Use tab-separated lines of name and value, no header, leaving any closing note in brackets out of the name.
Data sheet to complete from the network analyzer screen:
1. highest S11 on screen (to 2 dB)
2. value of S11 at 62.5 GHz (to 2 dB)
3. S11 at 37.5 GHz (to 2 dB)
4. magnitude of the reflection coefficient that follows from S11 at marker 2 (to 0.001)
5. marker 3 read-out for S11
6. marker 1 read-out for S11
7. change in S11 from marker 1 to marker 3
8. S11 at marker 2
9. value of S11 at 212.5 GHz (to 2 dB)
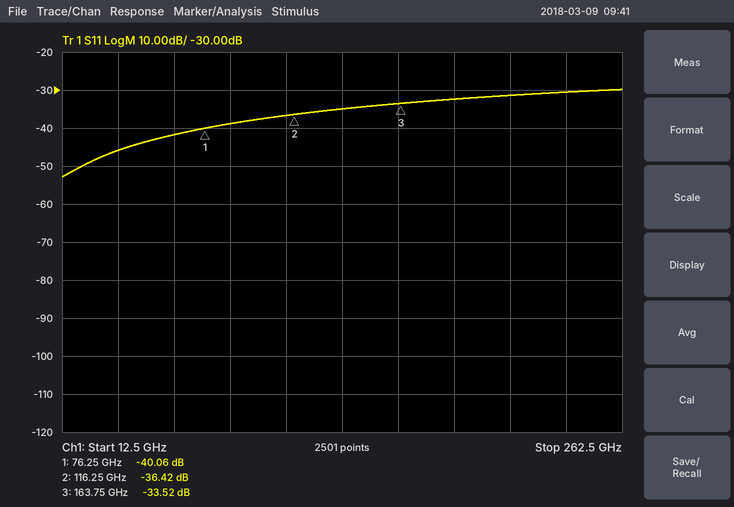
highest S11 on screen	-30 dB
value of S11 at 62.5 GHz	-42 dB
S11 at 37.5 GHz	-46 dB
magnitude of the reflection coefficient that follows from S11 at marker 2	0.015
marker 3 read-out for S11	-33.52 dB
marker 1 read-out for S11	-40.06 dB
change in S11 from marker 1 to marker 3	6.54 dB
S11 at marker 2	-36.42 dB
value of S11 at 212.5 GHz	-32 dB
